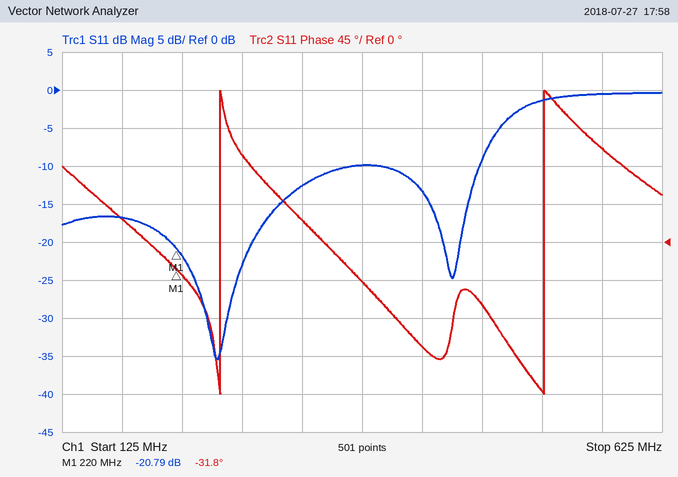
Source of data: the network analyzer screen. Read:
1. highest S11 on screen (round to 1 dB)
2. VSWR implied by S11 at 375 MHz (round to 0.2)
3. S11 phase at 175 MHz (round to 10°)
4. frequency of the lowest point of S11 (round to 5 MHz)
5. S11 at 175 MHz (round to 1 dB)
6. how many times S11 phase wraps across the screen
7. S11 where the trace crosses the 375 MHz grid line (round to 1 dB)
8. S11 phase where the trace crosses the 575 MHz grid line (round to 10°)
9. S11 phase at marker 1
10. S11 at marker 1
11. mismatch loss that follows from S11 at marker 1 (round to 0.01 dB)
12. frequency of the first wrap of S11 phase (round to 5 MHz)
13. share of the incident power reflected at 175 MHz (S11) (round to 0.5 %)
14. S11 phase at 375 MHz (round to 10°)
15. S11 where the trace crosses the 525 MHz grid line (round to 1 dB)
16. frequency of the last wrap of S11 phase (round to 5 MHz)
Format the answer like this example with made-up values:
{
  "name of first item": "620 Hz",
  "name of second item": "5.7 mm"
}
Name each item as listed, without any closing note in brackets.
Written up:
{
  "highest S11 on screen": "0 dB",
  "VSWR implied by S11 at 375 MHz": "2.0",
  "S11 phase at 175 MHz": "30°",
  "frequency of the lowest point of S11": "255 MHz",
  "S11 at 175 MHz": "-17 dB",
  "how many times S11 phase wraps across the screen": "2",
  "S11 where the trace crosses the 375 MHz grid line": "-10 dB",
  "S11 phase where the trace crosses the 575 MHz grid line": "110°",
  "S11 phase at marker 1": "-31.8°",
  "S11 at marker 1": "-20.79 dB",
  "mismatch loss that follows from S11 at marker 1": "0.04 dB",
  "frequency of the first wrap of S11 phase": "255 MHz",
  "share of the incident power reflected at 175 MHz (S11)": "2.0 %",
  "S11 phase at 375 MHz": "-50°",
  "S11 where the trace crosses the 525 MHz grid line": "-1 dB",
  "frequency of the last wrap of S11 phase": "525 MHz"
}
